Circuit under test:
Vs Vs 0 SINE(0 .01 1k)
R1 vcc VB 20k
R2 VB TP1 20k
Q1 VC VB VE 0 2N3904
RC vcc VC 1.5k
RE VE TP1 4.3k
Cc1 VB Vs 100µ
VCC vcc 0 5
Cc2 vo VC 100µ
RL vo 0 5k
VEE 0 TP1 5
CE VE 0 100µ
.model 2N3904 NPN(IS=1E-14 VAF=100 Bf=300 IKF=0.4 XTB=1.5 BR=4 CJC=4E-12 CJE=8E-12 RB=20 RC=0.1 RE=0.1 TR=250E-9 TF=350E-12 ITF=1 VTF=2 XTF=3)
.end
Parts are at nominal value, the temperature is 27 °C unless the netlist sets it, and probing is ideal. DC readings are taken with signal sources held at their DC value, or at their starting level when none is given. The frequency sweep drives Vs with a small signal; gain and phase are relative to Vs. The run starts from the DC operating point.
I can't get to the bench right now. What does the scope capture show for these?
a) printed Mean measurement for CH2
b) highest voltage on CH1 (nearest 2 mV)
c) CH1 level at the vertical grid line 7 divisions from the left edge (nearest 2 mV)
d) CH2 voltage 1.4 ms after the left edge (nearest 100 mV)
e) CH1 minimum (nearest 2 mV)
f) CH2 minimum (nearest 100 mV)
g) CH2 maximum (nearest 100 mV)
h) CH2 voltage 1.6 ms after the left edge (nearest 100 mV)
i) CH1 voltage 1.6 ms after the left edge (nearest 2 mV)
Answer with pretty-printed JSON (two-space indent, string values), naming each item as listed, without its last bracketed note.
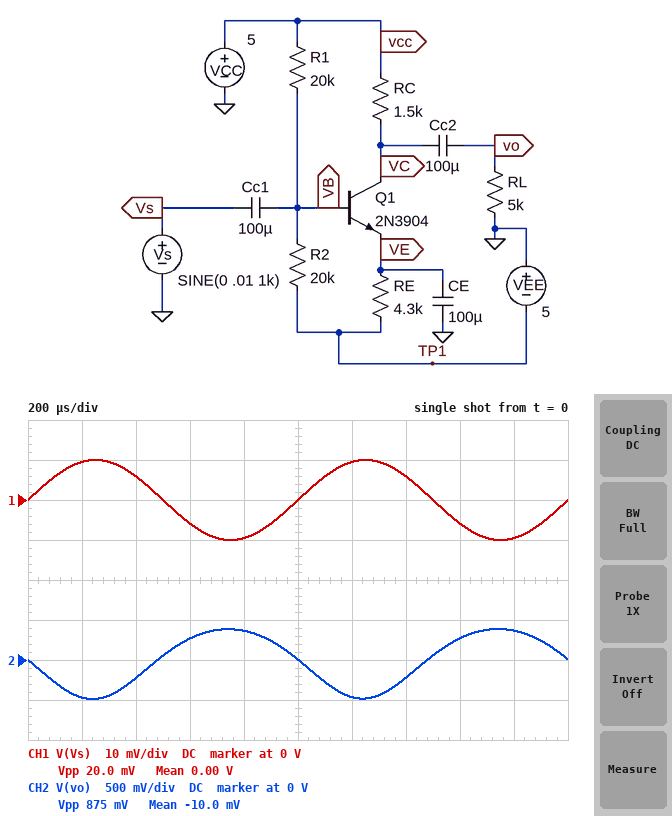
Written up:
{
  "printed Mean measurement for CH2": "-10.0 mV",
  "highest voltage on CH1": "10 mV",
  "CH1 level at the vertical grid line 7 divisions from the left edge": "6 mV",
  "CH2 voltage 1.4 ms after the left edge": "-200 mV",
  "CH1 minimum": "-10 mV",
  "CH2 minimum": "-500 mV",
  "CH2 maximum": "400 mV",
  "CH2 voltage 1.6 ms after the left edge": "300 mV",
  "CH1 voltage 1.6 ms after the left edge": "-6 mV"
}
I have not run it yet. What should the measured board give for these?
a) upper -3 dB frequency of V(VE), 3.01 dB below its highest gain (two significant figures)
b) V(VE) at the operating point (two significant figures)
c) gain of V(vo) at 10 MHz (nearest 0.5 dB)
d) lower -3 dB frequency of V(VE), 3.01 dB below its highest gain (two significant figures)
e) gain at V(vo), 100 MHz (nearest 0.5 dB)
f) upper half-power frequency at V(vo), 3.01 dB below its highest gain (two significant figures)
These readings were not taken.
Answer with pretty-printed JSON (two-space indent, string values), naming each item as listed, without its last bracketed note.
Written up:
{
  "upper -3 dB frequency of V(VE), 3.01 dB below its highest gain": "61 Hz",
  "V(VE) at the operating point": "-690 mV",
  "gain of V(vo) at 10 MHz": "32.5 dB",
  "lower -3 dB frequency of V(VE), 3.01 dB below its highest gain": "160 mHz",
  "gain at V(vo), 100 MHz": "22.5 dB",
  "upper half-power frequency at V(vo), 3.01 dB below its highest gain": "33 MHz"
}
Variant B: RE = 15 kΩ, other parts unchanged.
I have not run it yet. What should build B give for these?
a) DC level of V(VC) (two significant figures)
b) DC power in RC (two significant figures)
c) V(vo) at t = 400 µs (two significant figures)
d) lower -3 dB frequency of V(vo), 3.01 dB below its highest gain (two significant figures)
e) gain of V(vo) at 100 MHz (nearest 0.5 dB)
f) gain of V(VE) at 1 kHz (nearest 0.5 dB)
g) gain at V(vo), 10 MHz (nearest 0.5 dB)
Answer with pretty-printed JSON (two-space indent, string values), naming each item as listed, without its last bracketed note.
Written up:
{
  "DC level of V(VC)": "4.6 V",
  "DC power in RC": "130 µW",
  "V(vo) at t = 400 µs": "-79 mV",
  "lower -3 dB frequency of V(vo), 3.01 dB below its highest gain": "18 Hz",
  "gain of V(vo) at 100 MHz": "15.5 dB",
  "gain of V(VE) at 1 kHz": "-35.0 dB",
  "gain at V(vo), 10 MHz": "22.0 dB"
}
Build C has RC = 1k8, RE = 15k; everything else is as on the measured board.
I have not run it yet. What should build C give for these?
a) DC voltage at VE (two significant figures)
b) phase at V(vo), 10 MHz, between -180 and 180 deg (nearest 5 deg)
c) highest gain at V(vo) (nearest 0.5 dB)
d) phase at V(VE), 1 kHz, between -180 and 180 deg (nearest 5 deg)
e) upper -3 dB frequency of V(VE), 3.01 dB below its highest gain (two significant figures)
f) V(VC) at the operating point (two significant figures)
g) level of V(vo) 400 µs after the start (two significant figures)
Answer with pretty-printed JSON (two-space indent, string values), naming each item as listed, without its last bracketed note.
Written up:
{
  "DC voltage at VE": "-630 mV",
  "phase at V(vo), 10 MHz, between -180 and 180 deg": "165 deg",
  "highest gain at V(vo)": "23.5 dB",
  "phase at V(VE), 1 kHz, between -180 and 180 deg": "-90 deg",
  "upper -3 dB frequency of V(VE), 3.01 dB below its highest gain": "18 Hz",
  "V(VC) at the operating point": "4.5 V",
  "level of V(vo) 400 µs after the start": "-90 mV"
}
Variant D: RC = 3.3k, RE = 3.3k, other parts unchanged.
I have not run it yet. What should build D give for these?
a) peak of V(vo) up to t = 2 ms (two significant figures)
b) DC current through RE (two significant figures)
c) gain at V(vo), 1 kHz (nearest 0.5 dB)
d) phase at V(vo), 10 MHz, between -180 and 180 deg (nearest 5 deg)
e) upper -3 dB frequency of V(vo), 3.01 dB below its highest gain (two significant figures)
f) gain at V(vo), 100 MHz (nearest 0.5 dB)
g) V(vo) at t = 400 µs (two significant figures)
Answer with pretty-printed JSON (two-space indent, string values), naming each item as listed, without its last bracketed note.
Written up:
{
  "peak of V(vo) up to t = 2 ms": "860 mV",
  "DC current through RE": "1.3 mA",
  "gain at V(vo), 1 kHz": "39.5 dB",
  "phase at V(vo), 10 MHz, between -180 and 180 deg": "140 deg",
  "upper -3 dB frequency of V(vo), 3.01 dB below its highest gain": "13 MHz",
  "gain at V(vo), 100 MHz": "21.5 dB",
  "V(vo) at t = 400 µs": "-460 mV"
}
